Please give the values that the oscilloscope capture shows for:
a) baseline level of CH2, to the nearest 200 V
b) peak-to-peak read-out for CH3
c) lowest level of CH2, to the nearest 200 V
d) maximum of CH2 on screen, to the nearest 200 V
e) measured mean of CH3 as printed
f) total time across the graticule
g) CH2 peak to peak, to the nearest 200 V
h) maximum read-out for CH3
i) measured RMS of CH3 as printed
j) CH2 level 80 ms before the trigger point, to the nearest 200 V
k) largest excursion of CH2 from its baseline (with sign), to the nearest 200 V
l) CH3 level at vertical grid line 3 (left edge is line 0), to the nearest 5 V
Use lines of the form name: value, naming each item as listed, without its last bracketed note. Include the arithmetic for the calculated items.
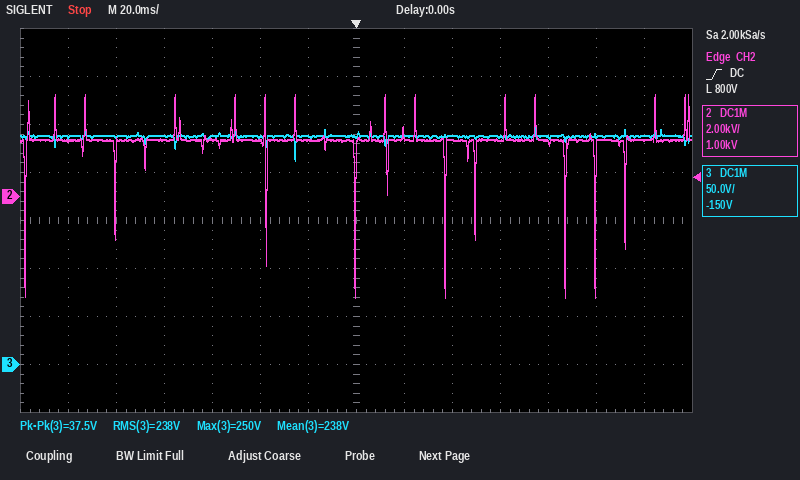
baseline level of CH2, to the nearest 200 V: 2.4 kV
peak-to-peak read-out for CH3: 37.5 V
lowest level of CH2, to the nearest 200 V: -4.2 kV
maximum of CH2 on screen, to the nearest 200 V: 4.2 kV
measured mean of CH3 as printed: 238 V
total time across the graticule: 280 ms
CH2 peak to peak, to the nearest 200 V: 4.2 kV − (-4.2 kV) = 8.4 kV
maximum read-out for CH3: 250 V
measured RMS of CH3 as printed: 238 V
CH2 level 80 ms before the trigger point, to the nearest 200 V: 2.4 kV
largest excursion of CH2 from its baseline (with sign), to the nearest 200 V: -4.2 kV − (2.4 kV) = -6.6 kV
CH3 level at vertical grid line 3 (left edge is line 0), to the nearest 5 V: 240 V
